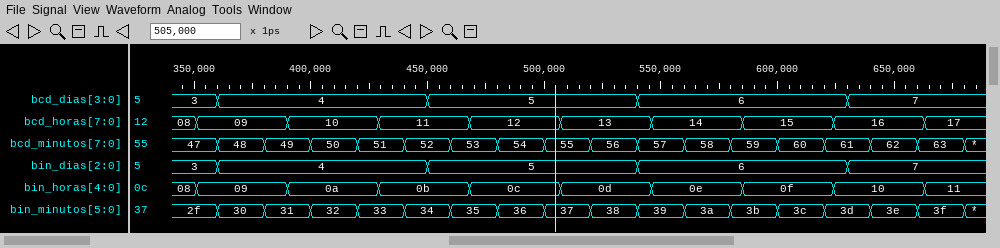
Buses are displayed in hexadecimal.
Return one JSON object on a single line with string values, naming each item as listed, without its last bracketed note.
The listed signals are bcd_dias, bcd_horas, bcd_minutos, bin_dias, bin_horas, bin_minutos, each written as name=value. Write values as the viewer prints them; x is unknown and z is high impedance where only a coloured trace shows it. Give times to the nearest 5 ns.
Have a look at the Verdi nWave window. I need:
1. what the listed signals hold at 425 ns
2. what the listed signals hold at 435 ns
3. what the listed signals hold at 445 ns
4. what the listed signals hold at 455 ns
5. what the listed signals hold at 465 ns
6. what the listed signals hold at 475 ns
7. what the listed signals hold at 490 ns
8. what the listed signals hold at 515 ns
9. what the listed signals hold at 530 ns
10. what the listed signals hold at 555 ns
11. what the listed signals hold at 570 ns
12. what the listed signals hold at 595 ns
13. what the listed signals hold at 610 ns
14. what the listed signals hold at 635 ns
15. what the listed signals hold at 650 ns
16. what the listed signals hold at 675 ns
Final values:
{"what the listed signals hold at 425 ns": "bcd_dias=4, bcd_horas=10, bcd_minutos=51, bin_dias=4, bin_horas=0a, bin_minutos=33", "what the listed signals hold at 435 ns": "bcd_dias=4, bcd_horas=11, bcd_minutos=51, bin_dias=4, bin_horas=0b, bin_minutos=33", "what the listed signals hold at 445 ns": "bcd_dias=4, bcd_horas=11, bcd_minutos=52, bin_dias=4, bin_horas=0b, bin_minutos=34", "what the listed signals hold at 455 ns": "bcd_dias=5, bcd_horas=11, bcd_minutos=52, bin_dias=5, bin_horas=0b, bin_minutos=34", "what the listed signals hold at 465 ns": "bcd_dias=5, bcd_horas=11, bcd_minutos=53, bin_dias=5, bin_horas=0b, bin_minutos=35", "what the listed signals hold at 475 ns": "bcd_dias=5, bcd_horas=12, bcd_minutos=53, bin_dias=5, bin_horas=0c, bin_minutos=35", "what the listed signals hold at 490 ns": "bcd_dias=5, bcd_horas=12, bcd_minutos=54, bin_dias=5, bin_horas=0c, bin_minutos=36", "what the listed signals hold at 515 ns": "bcd_dias=5, bcd_horas=13, bcd_minutos=55, bin_dias=5, bin_horas=0d, bin_minutos=37", "what the listed signals hold at 530 ns": "bcd_dias=5, bcd_horas=13, bcd_minutos=56, bin_dias=5, bin_horas=0d, bin_minutos=38", "what the listed signals hold at 555 ns": "bcd_dias=6, bcd_horas=14, bcd_minutos=57, bin_dias=6, bin_horas=0e, bin_minutos=39", "what the listed signals hold at 570 ns": "bcd_dias=6, bcd_horas=14, bcd_minutos=58, bin_dias=6, bin_horas=0e, bin_minutos=3a", "what the listed signals hold at 595 ns": "bcd_dias=6, bcd_horas=15, bcd_minutos=59, bin_dias=6, bin_horas=0f, bin_minutos=3b", "what the listed signals hold at 610 ns": "bcd_dias=6, bcd_horas=15, bcd_minutos=60, bin_dias=6, bin_horas=0f, bin_minutos=3c", "what the listed signals hold at 635 ns": "bcd_dias=7, bcd_horas=16, bcd_minutos=61, bin_dias=7, bin_horas=10, bin_minutos=3d", "what the listed signals hold at 650 ns": "bcd_dias=7, bcd_horas=16, bcd_minutos=62, bin_dias=7, bin_horas=10, bin_minutos=3e", "what the listed signals hold at 675 ns": "bcd_dias=7, bcd_horas=17, bcd_minutos=63, bin_dias=7, bin_horas=11, bin_minutos=3f"}
